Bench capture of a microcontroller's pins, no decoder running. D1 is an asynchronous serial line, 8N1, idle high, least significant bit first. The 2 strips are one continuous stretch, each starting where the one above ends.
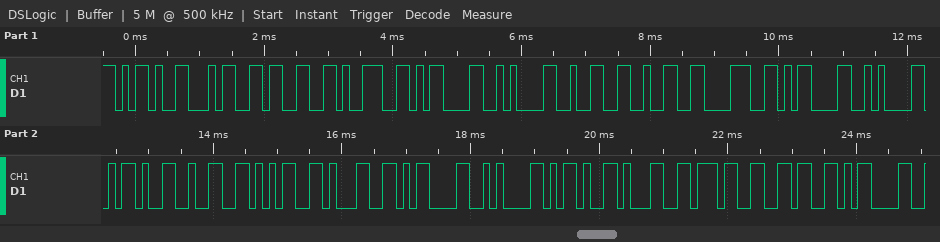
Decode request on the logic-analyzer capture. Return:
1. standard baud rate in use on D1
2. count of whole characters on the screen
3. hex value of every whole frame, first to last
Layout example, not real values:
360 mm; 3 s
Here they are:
9600 baud; 22; 2D 34 33 39 0D 0A 32 32 38 0D 0A 2D 32 35 31 0D 0A 2D 31 37 36 0D
